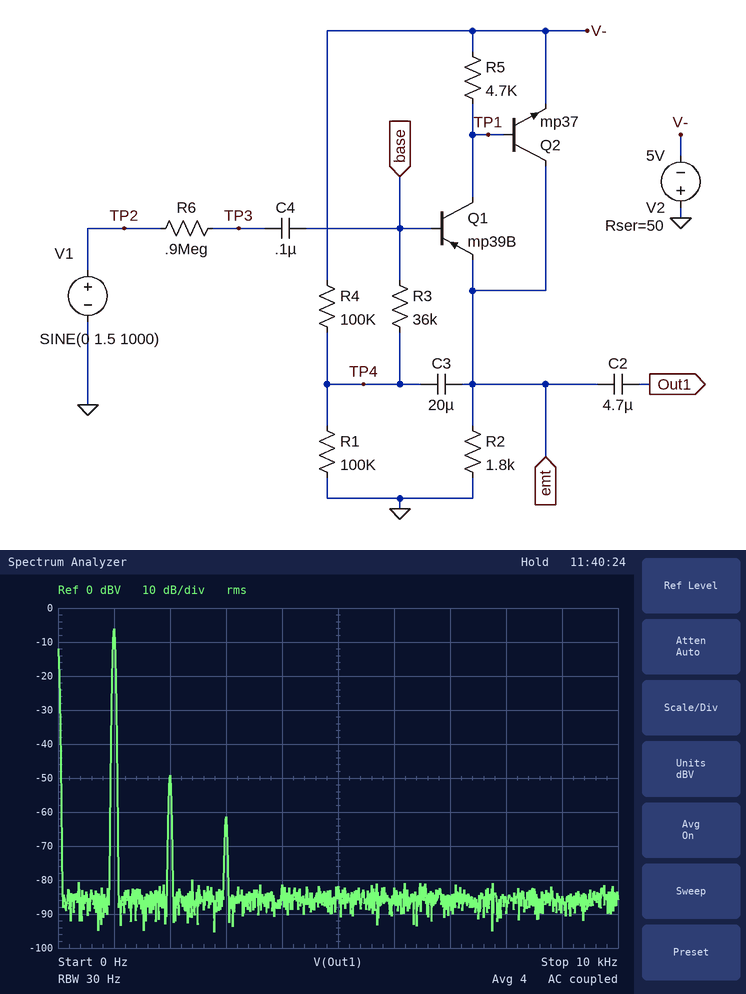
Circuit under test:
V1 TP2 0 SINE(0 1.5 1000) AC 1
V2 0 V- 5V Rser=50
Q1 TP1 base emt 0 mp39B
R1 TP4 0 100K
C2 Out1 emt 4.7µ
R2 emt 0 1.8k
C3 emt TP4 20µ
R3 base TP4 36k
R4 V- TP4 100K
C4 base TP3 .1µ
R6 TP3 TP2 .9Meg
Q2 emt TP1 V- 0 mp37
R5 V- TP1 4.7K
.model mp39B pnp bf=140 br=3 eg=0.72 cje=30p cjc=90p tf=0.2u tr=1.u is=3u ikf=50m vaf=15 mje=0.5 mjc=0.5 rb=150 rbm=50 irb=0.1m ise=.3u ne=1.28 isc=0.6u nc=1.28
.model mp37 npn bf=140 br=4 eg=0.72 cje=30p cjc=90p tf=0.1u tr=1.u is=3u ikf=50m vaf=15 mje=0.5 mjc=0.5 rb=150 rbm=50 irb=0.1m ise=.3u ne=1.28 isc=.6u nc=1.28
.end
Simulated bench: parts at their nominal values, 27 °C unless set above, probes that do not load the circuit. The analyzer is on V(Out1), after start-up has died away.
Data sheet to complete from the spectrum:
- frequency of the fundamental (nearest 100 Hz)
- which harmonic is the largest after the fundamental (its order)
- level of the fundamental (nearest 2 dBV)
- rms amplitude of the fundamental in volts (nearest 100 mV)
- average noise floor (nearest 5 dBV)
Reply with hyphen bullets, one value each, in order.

- 1.0 kHz
- 2
- -6 dBV
- 500 mV
- -85 dBV
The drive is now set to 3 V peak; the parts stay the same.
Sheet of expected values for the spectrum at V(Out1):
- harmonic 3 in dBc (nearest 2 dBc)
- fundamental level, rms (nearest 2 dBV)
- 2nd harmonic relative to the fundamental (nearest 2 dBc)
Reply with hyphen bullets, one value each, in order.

- -42 dBc
- 0 dBV
- -36 dBc
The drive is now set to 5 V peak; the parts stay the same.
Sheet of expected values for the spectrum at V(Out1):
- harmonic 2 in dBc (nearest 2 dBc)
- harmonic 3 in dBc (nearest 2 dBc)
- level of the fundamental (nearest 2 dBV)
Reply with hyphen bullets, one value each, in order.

- -28 dBc
- -30 dBc
- 4 dBV
